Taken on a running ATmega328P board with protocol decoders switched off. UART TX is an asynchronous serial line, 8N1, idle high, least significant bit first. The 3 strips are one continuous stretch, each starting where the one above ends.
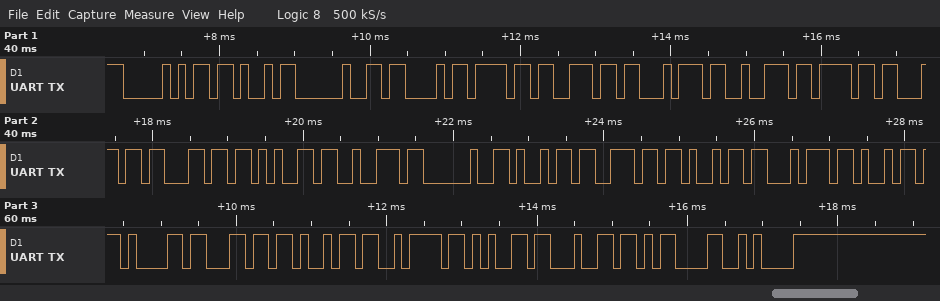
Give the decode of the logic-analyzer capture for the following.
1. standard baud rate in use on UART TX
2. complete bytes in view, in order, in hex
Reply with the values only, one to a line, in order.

9600 baud
50 4B 20 43 6F 6E 74 72 6F 6C 6C 65 72 20 69 6E 69 74 69 61 6C 69 7A 65 64 0D 0A
